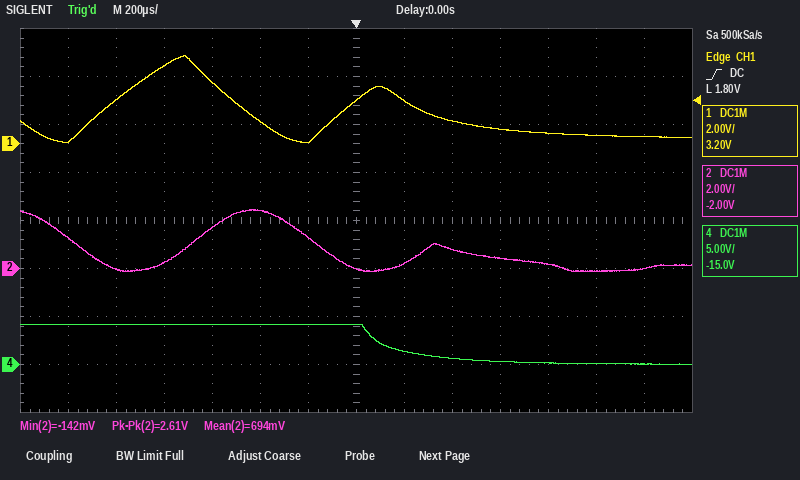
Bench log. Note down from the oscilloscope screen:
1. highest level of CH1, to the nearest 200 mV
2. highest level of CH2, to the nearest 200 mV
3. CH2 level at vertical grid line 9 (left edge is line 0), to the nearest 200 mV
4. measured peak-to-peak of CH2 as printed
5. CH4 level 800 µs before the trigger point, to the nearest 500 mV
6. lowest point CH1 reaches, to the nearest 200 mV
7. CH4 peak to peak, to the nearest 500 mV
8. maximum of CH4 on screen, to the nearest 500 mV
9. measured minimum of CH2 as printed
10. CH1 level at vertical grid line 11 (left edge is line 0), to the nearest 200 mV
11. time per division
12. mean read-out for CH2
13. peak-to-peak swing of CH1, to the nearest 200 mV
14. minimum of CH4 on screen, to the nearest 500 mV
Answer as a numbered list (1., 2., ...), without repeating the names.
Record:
1. 3.6 V
2. 2.4 V
3. 800 mV
4. 2.61 V
5. 4.0 V
6. 0.0 V
7. 4.0 V
8. 4.0 V
9. -142 mV
10. 400 mV
11. 200 µs
12. 694 mV
13. 3.6 V
14. 0.0 V
